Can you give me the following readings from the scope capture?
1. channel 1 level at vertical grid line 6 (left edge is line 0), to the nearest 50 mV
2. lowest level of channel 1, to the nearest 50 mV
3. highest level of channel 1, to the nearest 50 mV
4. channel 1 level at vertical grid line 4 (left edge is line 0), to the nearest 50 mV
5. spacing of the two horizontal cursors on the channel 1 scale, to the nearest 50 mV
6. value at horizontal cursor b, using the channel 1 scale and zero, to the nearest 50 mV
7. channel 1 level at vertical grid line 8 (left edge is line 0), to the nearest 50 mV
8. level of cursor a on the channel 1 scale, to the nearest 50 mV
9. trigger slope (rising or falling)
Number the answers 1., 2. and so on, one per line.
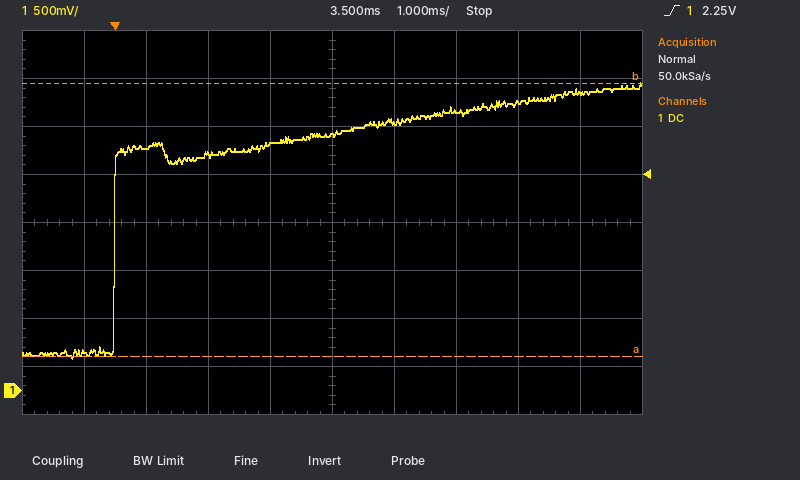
1. 2.80 V
2. 350 mV
3. 3.20 V
4. 2.55 V
5. 2.85 V
6. 3.20 V
7. 3.00 V
8. 350 mV
9. rising
